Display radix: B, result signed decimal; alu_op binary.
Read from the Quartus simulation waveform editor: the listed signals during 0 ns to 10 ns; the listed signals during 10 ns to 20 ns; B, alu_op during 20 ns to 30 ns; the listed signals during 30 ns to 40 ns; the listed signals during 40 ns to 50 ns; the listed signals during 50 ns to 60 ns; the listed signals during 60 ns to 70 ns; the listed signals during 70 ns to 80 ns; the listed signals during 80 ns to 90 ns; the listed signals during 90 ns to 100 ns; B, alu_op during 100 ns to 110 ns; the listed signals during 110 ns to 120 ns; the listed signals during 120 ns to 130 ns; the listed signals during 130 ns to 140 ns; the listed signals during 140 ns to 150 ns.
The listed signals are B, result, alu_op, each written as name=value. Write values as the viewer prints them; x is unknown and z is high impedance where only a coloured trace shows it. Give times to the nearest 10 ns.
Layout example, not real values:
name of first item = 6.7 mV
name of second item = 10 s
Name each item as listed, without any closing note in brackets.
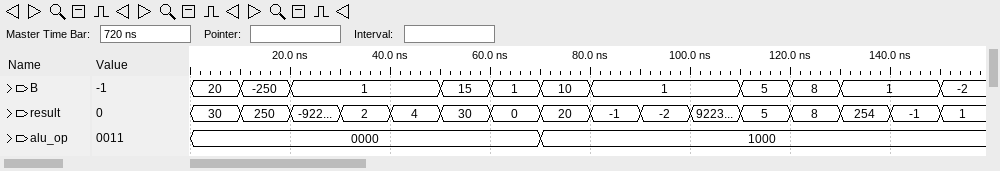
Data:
the listed signals during 0 ns to 10 ns = B=20, result=30, alu_op=0000
the listed signals during 10 ns to 20 ns = B=-250, result=250, alu_op=0000
B, alu_op during 20 ns to 30 ns = B=1, alu_op=0000
the listed signals during 30 ns to 40 ns = B=1, result=2, alu_op=0000
the listed signals during 40 ns to 50 ns = B=1, result=4, alu_op=0000
the listed signals during 50 ns to 60 ns = B=15, result=30, alu_op=0000
the listed signals during 60 ns to 70 ns = B=1, result=0, alu_op=0000
the listed signals during 70 ns to 80 ns = B=10, result=20, alu_op=1000
the listed signals during 80 ns to 90 ns = B=1, result=-1, alu_op=1000
the listed signals during 90 ns to 100 ns = B=1, result=-2, alu_op=1000
B, alu_op during 100 ns to 110 ns = B=1, alu_op=1000
the listed signals during 110 ns to 120 ns = B=5, result=5, alu_op=1000
the listed signals during 120 ns to 130 ns = B=8, result=8, alu_op=1000
the listed signals during 130 ns to 140 ns = B=1, result=254, alu_op=1000
the listed signals during 140 ns to 150 ns = B=1, result=-1, alu_op=1000
